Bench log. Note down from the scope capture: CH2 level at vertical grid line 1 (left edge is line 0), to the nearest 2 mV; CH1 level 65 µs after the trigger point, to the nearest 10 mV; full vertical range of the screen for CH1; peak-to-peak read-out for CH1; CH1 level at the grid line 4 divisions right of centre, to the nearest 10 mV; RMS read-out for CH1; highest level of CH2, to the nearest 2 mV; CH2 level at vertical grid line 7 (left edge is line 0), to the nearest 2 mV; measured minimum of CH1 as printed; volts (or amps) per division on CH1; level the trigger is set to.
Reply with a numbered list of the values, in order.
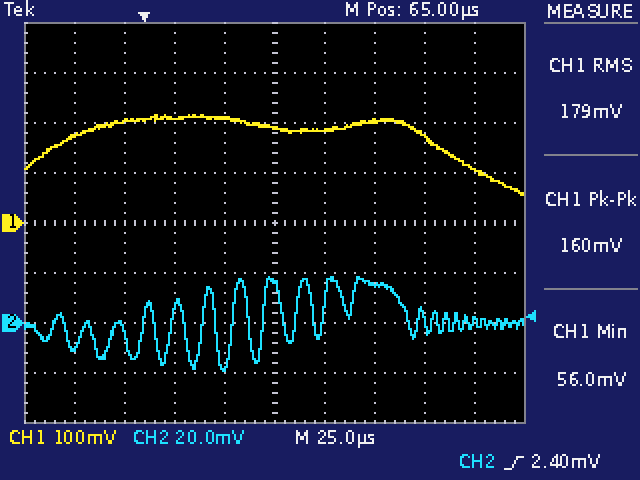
1. -10 mV
2. 190 mV
3. 800 mV
4. 160 mV
5. 110 mV
6. 179 mV
7. 18 mV
8. 16 mV
9. 56.0 mV
10. 100 mV
11. 2.40 mV
